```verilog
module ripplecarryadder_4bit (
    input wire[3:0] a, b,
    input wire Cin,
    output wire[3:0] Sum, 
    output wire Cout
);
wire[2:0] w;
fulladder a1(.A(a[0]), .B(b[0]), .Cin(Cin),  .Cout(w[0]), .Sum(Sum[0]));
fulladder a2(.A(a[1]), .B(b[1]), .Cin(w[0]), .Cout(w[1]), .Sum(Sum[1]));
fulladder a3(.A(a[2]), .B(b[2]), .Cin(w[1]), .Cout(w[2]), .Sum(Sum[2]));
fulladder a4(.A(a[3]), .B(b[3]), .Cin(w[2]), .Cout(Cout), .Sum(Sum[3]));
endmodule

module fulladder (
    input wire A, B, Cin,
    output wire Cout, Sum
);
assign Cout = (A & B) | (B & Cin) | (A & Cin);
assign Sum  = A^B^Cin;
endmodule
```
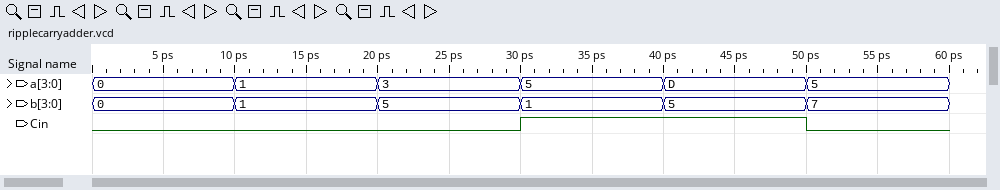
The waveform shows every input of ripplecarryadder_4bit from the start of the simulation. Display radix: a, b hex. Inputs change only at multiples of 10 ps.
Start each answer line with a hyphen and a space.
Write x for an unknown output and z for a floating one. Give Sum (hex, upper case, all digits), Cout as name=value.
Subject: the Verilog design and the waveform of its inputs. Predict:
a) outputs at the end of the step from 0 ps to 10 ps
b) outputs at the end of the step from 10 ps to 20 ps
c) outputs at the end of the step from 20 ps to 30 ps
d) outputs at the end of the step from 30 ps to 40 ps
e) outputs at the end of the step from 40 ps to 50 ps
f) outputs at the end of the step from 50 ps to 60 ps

- Sum=0, Cout=0
- Sum=2, Cout=0
- Sum=8, Cout=0
- Sum=7, Cout=0
- Sum=3, Cout=1
- Sum=C, Cout=0
